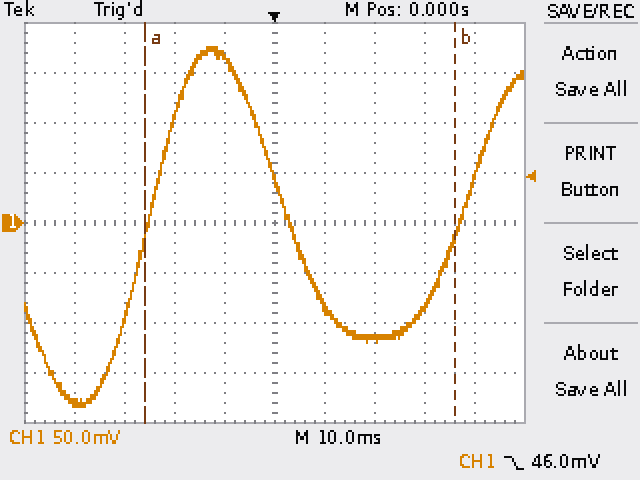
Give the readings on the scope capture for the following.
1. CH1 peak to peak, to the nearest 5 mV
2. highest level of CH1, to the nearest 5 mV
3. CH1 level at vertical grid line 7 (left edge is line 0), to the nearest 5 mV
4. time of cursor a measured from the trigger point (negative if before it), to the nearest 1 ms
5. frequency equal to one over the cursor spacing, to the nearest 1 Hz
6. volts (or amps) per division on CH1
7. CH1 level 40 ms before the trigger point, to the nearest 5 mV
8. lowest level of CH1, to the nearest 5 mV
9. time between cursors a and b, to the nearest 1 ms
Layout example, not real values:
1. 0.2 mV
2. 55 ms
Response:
1. 360 mV
2. 175 mV
3. -115 mV
4. -26 ms
5. 16 Hz
6. 50 mV
7. -180 mV
8. -185 mV
9. 62 ms
